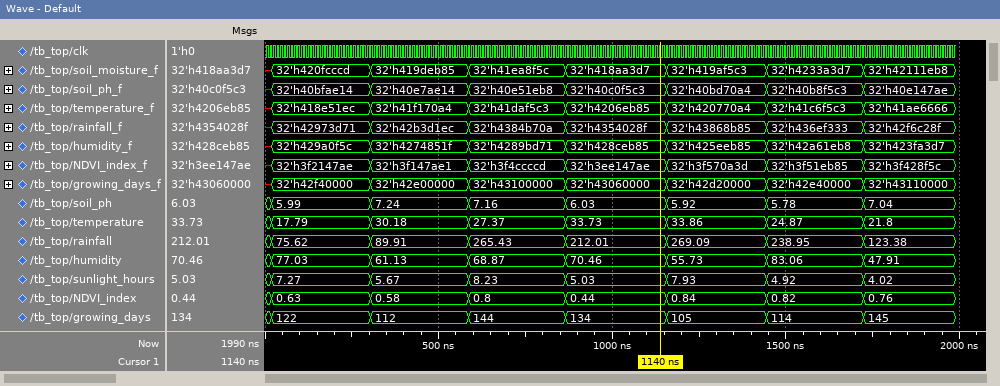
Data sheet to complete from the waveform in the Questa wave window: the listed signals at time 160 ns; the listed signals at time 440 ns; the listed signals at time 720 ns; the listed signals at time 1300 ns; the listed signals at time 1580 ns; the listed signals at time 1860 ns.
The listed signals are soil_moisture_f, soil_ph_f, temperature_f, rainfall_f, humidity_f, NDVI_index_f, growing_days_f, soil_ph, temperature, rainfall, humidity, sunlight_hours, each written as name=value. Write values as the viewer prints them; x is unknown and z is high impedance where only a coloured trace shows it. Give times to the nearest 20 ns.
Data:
soil_moisture_f=32'h420fcccd, soil_ph_f=32'h40bfae14, temperature_f=32'h418e51ec, rainfall_f=32'h42973d71, humidity_f=32'h429a0f5c, NDVI_index_f=32'h3f2147ae, growing_days_f=32'h42f40000, soil_ph=5.99, temperature=17.79, rainfall=75.62, humidity=77.03, sunlight_hours=7.27
soil_moisture_f=32'h419deb85, soil_ph_f=32'h40e7ae14, temperature_f=32'h41f170a4, rainfall_f=32'h42b3d1ec, humidity_f=32'h4274851f, NDVI_index_f=32'h3f147ae1, growing_days_f=32'h42e00000, soil_ph=7.24, temperature=30.18, rainfall=89.91, humidity=61.13, sunlight_hours=5.67
soil_moisture_f=32'h41ea8f5c, soil_ph_f=32'h40e51eb8, temperature_f=32'h41daf5c3, rainfall_f=32'h4384b70a, humidity_f=32'h4289bd71, NDVI_index_f=32'h3f4ccccd, growing_days_f=32'h43100000, soil_ph=7.16, temperature=27.37, rainfall=265.43, humidity=68.87, sunlight_hours=8.23
soil_moisture_f=32'h419af5c3, soil_ph_f=32'h40bd70a4, temperature_f=32'h420770a4, rainfall_f=32'h43868b85, humidity_f=32'h425eeb85, NDVI_index_f=32'h3f570a3d, growing_days_f=32'h42d20000, soil_ph=5.92, temperature=33.86, rainfall=269.09, humidity=55.73, sunlight_hours=7.93
soil_moisture_f=32'h4233a3d7, soil_ph_f=32'h40b8f5c3, temperature_f=32'h41c6f5c3, rainfall_f=32'h436ef333, humidity_f=32'h42a61eb8, NDVI_index_f=32'h3f51eb85, growing_days_f=32'h42e40000, soil_ph=5.78, temperature=24.87, rainfall=238.95, humidity=83.06, sunlight_hours=4.92
soil_moisture_f=32'h42111eb8, soil_ph_f=32'h40e147ae, temperature_f=32'h41ae6666, rainfall_f=32'h42f6c28f, humidity_f=32'h423fa3d7, NDVI_index_f=32'h3f428f5c, growing_days_f=32'h43110000, soil_ph=7.04, temperature=21.8, rainfall=123.38, humidity=47.91, sunlight_hours=4.02
